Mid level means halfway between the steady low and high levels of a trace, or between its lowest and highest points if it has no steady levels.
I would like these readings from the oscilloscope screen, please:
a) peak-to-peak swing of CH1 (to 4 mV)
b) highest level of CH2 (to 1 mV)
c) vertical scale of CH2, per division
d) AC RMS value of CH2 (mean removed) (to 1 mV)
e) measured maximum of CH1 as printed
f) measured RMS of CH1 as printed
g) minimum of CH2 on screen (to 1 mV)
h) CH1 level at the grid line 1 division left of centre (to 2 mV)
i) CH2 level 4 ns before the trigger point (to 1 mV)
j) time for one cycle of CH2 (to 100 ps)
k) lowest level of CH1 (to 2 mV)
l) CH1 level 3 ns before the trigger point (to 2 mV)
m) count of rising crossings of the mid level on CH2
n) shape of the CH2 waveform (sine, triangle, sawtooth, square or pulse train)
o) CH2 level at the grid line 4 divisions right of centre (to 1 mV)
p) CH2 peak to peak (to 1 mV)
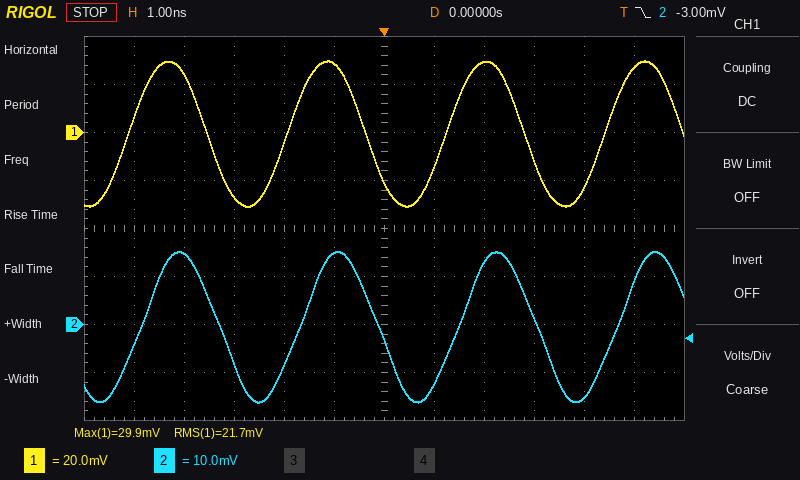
60 mV
15 mV
10 mV
11 mV
29.9 mV
21.7 mV
-16 mV
28 mV
15 mV
3.2 ns
-30 mV
-26 mV
4
sine
-15 mV
31 mV
